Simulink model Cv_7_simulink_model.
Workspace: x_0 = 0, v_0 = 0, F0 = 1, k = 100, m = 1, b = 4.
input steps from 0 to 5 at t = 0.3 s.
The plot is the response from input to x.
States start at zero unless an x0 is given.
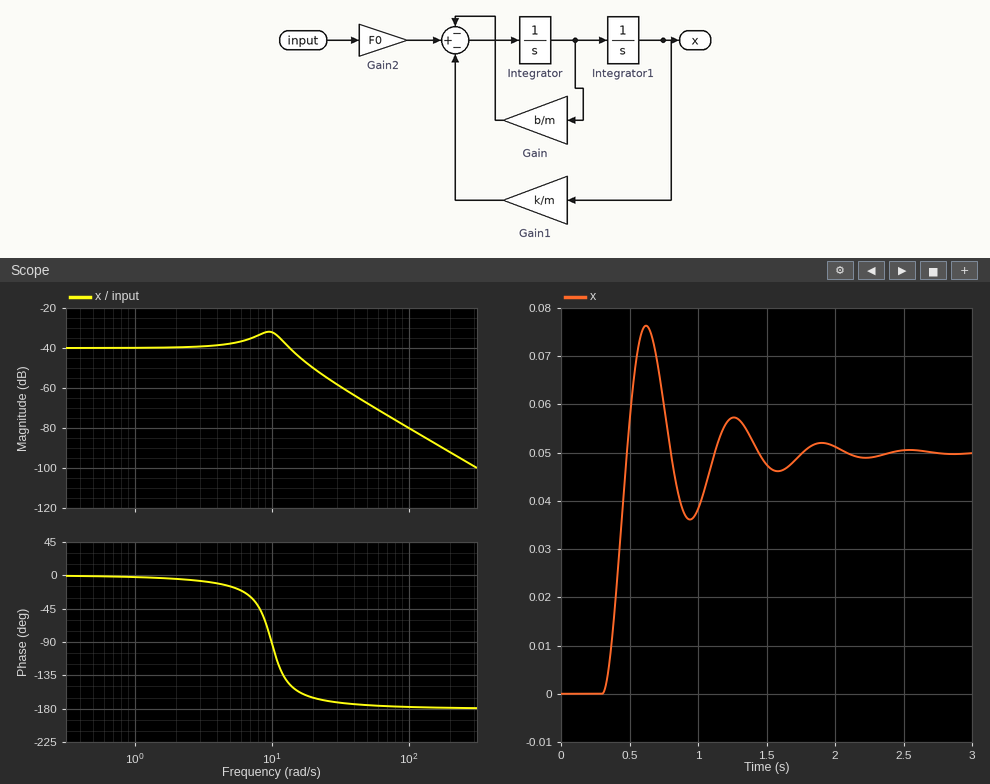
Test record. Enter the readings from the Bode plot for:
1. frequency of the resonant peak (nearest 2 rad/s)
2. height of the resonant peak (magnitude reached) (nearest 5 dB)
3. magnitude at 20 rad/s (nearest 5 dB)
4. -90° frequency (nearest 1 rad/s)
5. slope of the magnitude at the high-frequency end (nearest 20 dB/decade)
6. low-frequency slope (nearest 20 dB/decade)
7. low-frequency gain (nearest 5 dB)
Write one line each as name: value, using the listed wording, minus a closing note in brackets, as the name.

frequency of the resonant peak: 10 rad/s
height of the resonant peak (magnitude reached): -30 dB
magnitude at 20 rad/s: -50 dB
-90° frequency: 10 rad/s
slope of the magnitude at the high-frequency end: -40 dB/decade
low-frequency slope: 0 dB/decade
low-frequency gain: -40 dB
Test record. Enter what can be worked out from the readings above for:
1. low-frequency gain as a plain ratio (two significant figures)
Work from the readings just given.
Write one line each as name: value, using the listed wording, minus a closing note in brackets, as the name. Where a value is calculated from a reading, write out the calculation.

low-frequency gain as a plain ratio: 10^(-40 / 20) = 0.010
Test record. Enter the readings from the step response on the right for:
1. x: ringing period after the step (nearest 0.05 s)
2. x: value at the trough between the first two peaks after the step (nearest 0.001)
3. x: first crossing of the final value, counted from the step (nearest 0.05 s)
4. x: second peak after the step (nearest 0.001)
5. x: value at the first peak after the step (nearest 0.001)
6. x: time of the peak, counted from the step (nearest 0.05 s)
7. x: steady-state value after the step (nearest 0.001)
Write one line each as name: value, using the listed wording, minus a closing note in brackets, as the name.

x: ringing period after the step: 0.65 s
x: value at the trough between the first two peaks after the step: 0.036
x: first crossing of the final value, counted from the step: 0.20 s
x: second peak after the step: 0.057
x: value at the first peak after the step: 0.076
x: time of the peak, counted from the step: 0.30 s
x: steady-state value after the step: 0.050
